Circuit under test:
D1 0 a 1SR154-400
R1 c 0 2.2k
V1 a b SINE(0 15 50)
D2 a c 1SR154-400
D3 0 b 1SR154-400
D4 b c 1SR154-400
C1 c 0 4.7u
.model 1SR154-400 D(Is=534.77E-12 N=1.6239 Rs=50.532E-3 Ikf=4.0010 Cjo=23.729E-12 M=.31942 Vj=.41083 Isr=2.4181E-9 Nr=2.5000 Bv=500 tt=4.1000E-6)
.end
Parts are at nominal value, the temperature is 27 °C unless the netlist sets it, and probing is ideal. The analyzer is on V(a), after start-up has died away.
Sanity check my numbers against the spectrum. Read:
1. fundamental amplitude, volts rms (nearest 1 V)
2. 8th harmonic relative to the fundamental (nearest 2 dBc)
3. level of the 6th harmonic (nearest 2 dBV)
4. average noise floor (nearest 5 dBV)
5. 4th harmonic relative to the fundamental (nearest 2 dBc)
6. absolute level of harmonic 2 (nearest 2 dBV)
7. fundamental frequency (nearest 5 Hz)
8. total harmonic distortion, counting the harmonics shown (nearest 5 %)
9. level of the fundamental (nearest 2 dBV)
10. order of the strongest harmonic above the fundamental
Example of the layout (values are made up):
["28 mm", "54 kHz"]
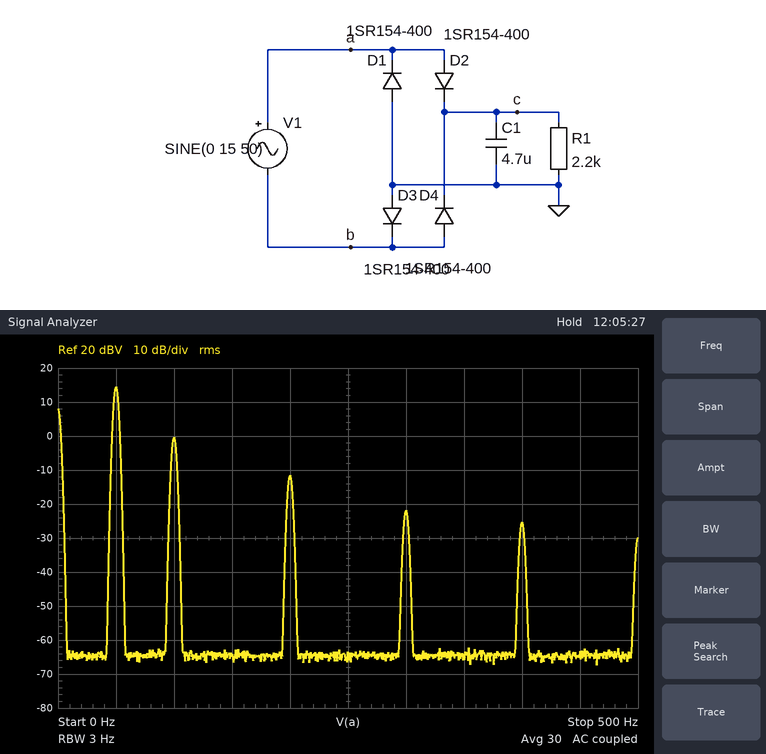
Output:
["5 V", "-40 dBc", "-22 dBV", "-65 dBV", "-26 dBc", "0 dBV", "50 Hz", "20 %", "14 dBV", "2"]
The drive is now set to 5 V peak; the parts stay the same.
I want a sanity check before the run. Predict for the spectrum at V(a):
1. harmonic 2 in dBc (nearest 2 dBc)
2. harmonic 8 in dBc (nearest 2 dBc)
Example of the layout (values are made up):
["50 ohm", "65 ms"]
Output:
["-16 dBc", "-42 dBc"]
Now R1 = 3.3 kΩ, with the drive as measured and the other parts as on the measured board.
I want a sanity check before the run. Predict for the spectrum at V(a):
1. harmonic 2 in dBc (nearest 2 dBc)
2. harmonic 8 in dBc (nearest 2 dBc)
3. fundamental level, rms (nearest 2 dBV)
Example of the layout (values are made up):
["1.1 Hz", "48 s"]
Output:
["-18 dBc", "-42 dBc", "14 dBV"]
